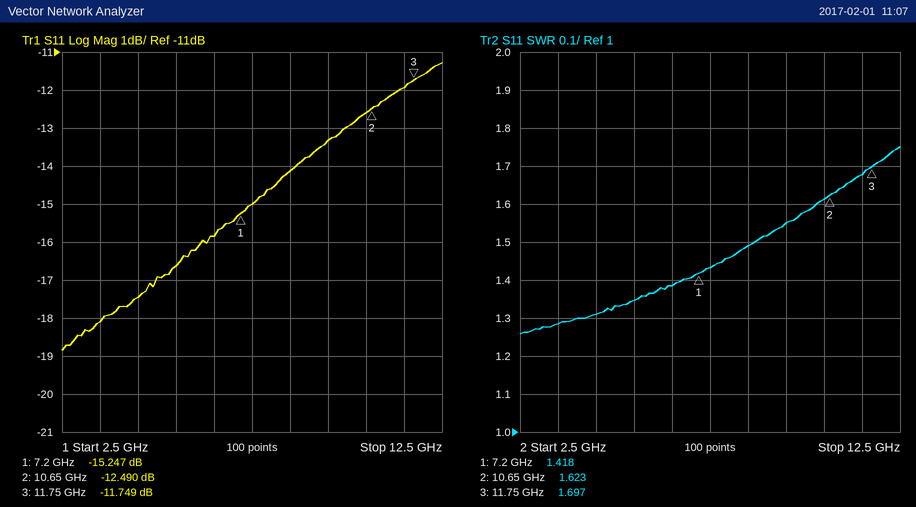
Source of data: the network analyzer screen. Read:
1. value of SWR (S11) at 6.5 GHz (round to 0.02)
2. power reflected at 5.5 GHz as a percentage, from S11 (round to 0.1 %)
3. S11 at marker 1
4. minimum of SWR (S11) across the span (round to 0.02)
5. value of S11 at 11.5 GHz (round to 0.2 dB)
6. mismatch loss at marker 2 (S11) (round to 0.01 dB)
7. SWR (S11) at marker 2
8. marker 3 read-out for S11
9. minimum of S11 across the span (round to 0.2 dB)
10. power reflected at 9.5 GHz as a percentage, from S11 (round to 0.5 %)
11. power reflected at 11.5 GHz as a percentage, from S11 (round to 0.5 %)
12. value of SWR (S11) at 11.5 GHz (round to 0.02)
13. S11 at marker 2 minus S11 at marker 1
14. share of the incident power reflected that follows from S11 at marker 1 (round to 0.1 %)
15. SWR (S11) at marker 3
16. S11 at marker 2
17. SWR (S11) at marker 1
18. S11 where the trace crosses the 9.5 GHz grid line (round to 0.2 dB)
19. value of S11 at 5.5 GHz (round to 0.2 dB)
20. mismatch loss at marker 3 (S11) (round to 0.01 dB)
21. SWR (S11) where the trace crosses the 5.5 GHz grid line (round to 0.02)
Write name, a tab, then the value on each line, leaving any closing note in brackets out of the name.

value of SWR (S11) at 6.5 GHz	1.38
power reflected at 5.5 GHz as a percentage, from S11	2.2 %
S11 at marker 1	-15.247 dB
minimum of SWR (S11) across the span	1.26
value of S11 at 11.5 GHz	-12.0 dB
mismatch loss at marker 2 (S11)	0.25 dB
SWR (S11) at marker 2	1.623
marker 3 read-out for S11	-11.749 dB
minimum of S11 across the span	-18.8 dB
power reflected at 9.5 GHz as a percentage, from S11	4.5 %
power reflected at 11.5 GHz as a percentage, from S11	6.5 %
value of SWR (S11) at 11.5 GHz	1.68
S11 at marker 2 minus S11 at marker 1	2.757 dB
share of the incident power reflected that follows from S11 at marker 1	3.0 %
SWR (S11) at marker 3	1.697
S11 at marker 2	-12.490 dB
SWR (S11) at marker 1	1.418
S11 where the trace crosses the 9.5 GHz grid line	-13.4 dB
value of S11 at 5.5 GHz	-16.6 dB
mismatch loss at marker 3 (S11)	0.30 dB
SWR (S11) where the trace crosses the 5.5 GHz grid line	1.34
